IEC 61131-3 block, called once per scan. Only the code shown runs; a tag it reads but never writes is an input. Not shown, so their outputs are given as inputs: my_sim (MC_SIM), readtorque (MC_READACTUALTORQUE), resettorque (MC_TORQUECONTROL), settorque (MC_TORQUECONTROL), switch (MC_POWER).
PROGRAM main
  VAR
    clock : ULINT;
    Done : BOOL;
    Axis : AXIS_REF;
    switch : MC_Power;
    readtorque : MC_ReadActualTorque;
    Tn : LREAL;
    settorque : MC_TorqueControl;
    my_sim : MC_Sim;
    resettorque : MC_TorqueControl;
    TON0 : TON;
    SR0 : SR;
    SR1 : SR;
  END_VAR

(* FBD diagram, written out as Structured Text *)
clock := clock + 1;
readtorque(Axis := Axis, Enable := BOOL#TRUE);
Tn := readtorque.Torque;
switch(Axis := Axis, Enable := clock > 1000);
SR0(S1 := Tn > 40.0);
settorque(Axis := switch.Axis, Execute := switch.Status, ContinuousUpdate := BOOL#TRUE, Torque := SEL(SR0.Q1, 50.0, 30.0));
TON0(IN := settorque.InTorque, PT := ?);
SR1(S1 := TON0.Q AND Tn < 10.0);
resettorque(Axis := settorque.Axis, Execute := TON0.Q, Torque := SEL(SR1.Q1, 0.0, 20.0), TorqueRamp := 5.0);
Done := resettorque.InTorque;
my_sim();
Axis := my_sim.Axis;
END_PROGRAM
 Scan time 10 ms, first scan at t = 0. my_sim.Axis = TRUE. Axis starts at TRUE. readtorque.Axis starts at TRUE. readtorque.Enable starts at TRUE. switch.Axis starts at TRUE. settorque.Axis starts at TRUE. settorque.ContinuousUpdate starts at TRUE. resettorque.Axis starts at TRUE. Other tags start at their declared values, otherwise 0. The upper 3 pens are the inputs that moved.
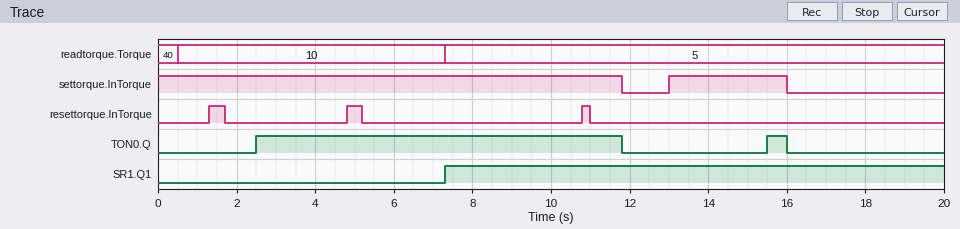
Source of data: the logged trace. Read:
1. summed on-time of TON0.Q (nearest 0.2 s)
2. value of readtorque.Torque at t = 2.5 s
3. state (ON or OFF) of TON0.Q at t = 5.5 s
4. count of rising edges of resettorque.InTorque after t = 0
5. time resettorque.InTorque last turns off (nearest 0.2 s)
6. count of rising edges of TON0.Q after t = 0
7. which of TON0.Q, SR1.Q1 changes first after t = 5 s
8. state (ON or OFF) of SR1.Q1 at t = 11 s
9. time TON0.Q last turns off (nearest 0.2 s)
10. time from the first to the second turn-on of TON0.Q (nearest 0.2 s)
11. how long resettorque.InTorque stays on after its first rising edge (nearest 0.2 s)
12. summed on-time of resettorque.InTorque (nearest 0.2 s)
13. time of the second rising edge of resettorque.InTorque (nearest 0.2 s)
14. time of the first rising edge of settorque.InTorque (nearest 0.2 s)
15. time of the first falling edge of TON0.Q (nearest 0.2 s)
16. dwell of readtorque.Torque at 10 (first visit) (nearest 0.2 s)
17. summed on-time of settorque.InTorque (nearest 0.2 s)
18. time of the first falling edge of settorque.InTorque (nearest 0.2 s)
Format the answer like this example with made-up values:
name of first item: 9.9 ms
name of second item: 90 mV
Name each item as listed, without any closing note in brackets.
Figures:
summed on-time of TON0.Q: 9.8 s
value of readtorque.Torque at t = 2.5 s: 10
state (ON or OFF) of TON0.Q at t = 5.5 s: ON
count of rising edges of resettorque.InTorque after t = 0: 3
time resettorque.InTorque last turns off: 11.0 s
count of rising edges of TON0.Q after t = 0: 2
which of TON0.Q, SR1.Q1 changes first after t = 5 s: SR1.Q1
state (ON or OFF) of SR1.Q1 at t = 11 s: ON
time TON0.Q last turns off: 16.0 s
time from the first to the second turn-on of TON0.Q: 13.0 s
how long resettorque.InTorque stays on after its first rising edge: 0.4 s
summed on-time of resettorque.InTorque: 1.0 s
time of the second rising edge of resettorque.InTorque: 4.8 s
time of the first rising edge of settorque.InTorque: 13.0 s
time of the first falling edge of TON0.Q: 11.8 s
dwell of readtorque.Torque at 10 (first visit): 6.8 s
summed on-time of settorque.InTorque: 14.8 s
time of the first falling edge of settorque.InTorque: 11.8 s
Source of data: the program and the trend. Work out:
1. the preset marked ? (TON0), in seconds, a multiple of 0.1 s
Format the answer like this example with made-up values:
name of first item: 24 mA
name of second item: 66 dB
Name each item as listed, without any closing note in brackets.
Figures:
the preset marked ? (TON0), in seconds, a multiple of 0.1 s: 2.5 s
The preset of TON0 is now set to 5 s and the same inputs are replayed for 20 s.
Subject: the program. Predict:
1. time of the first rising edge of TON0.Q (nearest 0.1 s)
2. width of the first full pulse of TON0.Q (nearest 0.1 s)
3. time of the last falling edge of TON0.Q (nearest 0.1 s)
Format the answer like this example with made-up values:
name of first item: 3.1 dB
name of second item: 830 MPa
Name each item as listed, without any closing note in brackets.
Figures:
time of the first rising edge of TON0.Q: 5.0 s
width of the first full pulse of TON0.Q: 6.8 s
time of the last falling edge of TON0.Q: 11.8 s
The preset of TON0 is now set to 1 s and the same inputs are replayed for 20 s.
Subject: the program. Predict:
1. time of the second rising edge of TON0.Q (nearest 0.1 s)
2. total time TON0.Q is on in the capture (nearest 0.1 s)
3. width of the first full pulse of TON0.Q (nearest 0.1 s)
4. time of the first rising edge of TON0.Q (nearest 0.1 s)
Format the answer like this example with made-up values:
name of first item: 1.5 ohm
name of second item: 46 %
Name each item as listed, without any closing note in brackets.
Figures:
time of the second rising edge of TON0.Q: 14.0 s
total time TON0.Q is on in the capture: 12.8 s
width of the first full pulse of TON0.Q: 10.8 s
time of the first rising edge of TON0.Q: 1.0 s
